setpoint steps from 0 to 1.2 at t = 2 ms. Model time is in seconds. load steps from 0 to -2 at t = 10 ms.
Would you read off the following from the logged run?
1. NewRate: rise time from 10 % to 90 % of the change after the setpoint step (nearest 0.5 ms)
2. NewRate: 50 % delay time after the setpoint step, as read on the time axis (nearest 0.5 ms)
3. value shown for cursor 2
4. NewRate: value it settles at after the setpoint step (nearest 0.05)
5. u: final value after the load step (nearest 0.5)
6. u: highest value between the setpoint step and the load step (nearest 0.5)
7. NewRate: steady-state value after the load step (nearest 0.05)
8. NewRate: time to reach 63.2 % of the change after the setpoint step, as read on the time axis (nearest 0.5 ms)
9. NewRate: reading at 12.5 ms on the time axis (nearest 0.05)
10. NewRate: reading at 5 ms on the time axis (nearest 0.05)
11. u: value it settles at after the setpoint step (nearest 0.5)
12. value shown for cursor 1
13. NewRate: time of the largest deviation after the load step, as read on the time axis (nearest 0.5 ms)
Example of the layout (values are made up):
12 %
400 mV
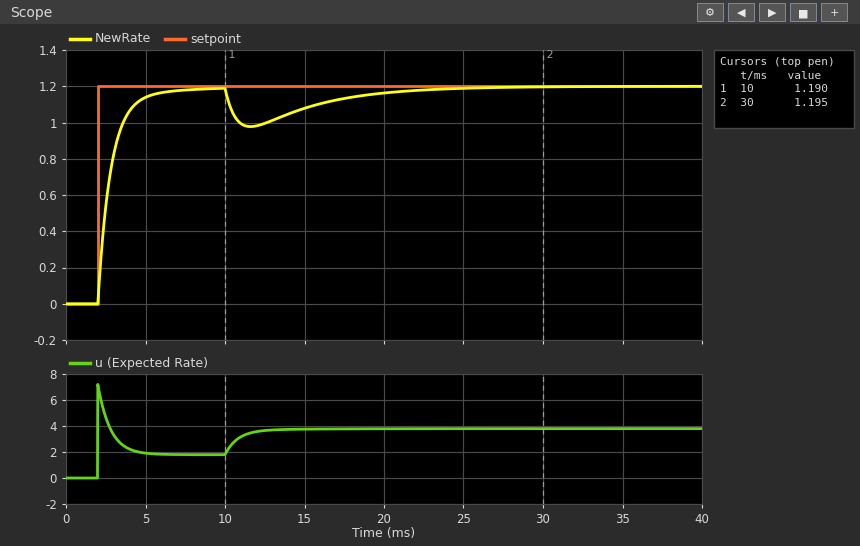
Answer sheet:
2.0 ms
2.5 ms
1.195
1.20
4.0
7.0
1.20
3.0 ms
1.00
1.15
2.0
1.190
11.5 ms
